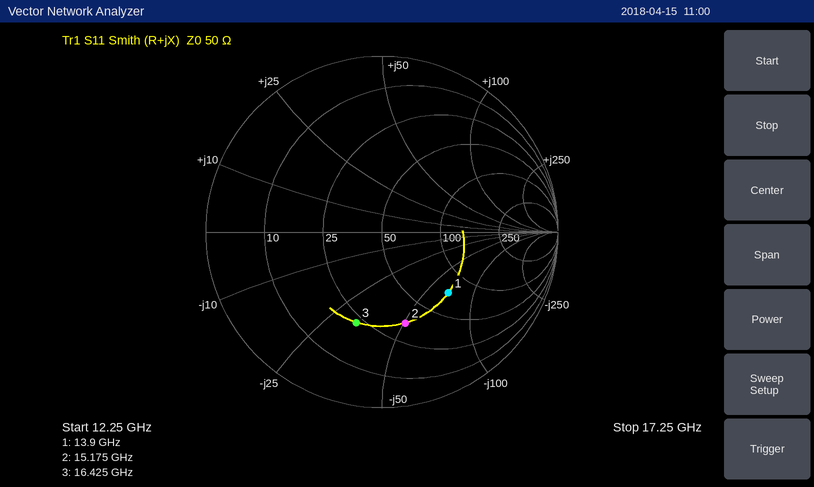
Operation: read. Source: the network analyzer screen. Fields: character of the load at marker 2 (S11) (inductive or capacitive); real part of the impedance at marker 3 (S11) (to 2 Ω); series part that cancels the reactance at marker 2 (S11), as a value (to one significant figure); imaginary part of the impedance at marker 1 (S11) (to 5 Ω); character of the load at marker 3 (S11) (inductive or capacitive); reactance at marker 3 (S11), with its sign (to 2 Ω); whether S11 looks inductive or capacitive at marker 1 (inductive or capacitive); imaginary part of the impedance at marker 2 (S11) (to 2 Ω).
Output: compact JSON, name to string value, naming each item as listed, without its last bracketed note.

{"character of the load at marker 2 (S11)": "capacitive", "real part of the impedance at marker 3 (S11)": "22 Ω", "series part that cancels the reactance at marker 2 (S11), as a value": "500 pH", "imaginary part of the impedance at marker 1 (S11)": "-70 Ω", "character of the load at marker 3 (S11)": "capacitive", "reactance at marker 3 (S11), with its sign": "-32 Ω", "whether S11 looks inductive or capacitive at marker 1": "capacitive", "imaginary part of the impedance at marker 2 (S11)": "-50 Ω"}
